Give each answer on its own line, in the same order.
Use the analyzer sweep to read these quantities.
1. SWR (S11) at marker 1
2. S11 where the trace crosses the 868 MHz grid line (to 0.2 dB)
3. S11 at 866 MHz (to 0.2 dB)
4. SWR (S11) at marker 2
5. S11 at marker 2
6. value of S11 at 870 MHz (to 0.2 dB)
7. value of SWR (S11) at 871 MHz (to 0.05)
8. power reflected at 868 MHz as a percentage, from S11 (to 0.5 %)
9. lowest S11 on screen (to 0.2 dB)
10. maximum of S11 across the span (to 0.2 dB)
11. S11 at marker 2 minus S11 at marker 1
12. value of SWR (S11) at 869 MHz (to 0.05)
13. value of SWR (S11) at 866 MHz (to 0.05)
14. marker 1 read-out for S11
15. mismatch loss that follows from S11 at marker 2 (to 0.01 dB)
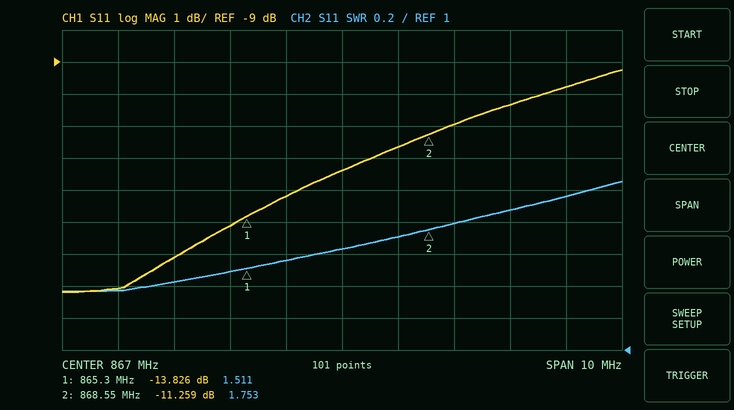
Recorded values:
1.511
-11.6 dB
-13.2 dB
1.753
-11.259 dB
-10.4 dB
1.95
7.0 %
-16.2 dB
-9.2 dB
2.567 dB
1.80
1.55
-13.826 dB
0.34 dB
